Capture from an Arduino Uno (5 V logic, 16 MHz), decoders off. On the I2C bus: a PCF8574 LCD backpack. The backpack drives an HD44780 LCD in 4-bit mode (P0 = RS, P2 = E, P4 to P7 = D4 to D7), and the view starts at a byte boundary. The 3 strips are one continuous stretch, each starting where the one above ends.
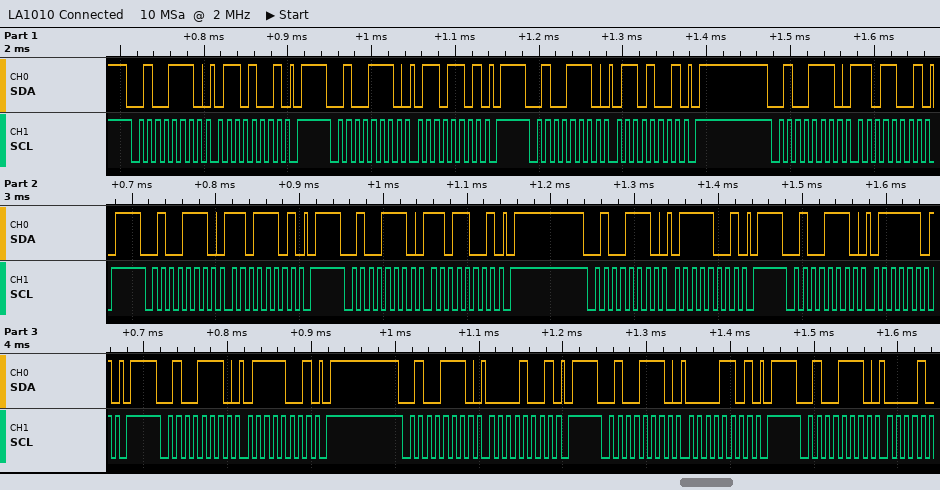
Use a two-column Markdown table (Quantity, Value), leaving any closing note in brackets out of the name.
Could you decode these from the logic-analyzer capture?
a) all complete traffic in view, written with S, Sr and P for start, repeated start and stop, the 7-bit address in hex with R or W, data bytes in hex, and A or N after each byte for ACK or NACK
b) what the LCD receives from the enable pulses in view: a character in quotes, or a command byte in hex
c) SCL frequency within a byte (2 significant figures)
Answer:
| Quantity | Value |
|---|---|
| all complete traffic in view, written with S, Sr and P for start, repeated start and stop, the 7-bit address in hex with R or W, data bytes in hex, and A or N after each byte for ACK or NACK | S 27W A 69 A P S 27W A 6D A P S 27W A 69 A P S 27W A D9 A P S 27W A DD A P S 27W A D9 A P S 27W A 79 A P S 27W A 7D A P S 27W A 79 A P S 27W A 09 A P S 27W A 0D A P S 27W A |
| what the LCD receives from the enable pulses in view: a character in quotes, or a command byte in hex | 'm' |
| SCL frequency within a byte | 100 kHz |
